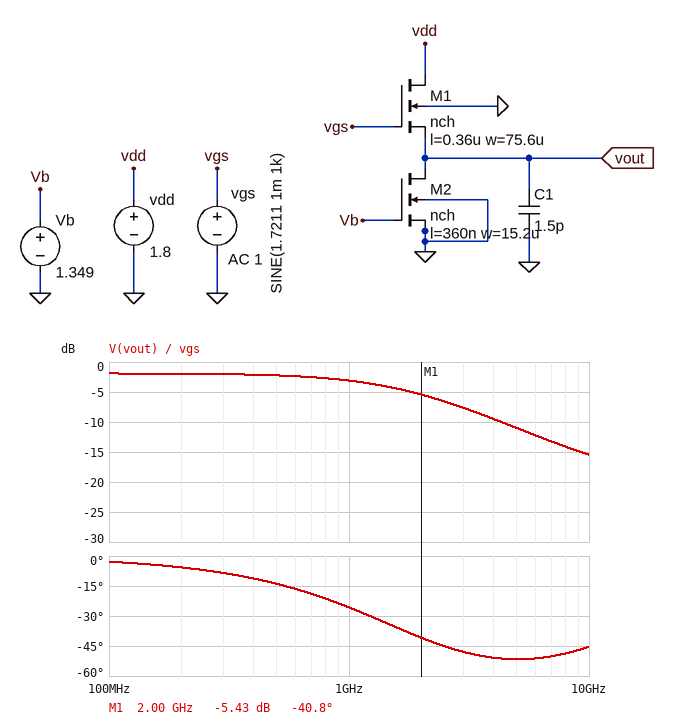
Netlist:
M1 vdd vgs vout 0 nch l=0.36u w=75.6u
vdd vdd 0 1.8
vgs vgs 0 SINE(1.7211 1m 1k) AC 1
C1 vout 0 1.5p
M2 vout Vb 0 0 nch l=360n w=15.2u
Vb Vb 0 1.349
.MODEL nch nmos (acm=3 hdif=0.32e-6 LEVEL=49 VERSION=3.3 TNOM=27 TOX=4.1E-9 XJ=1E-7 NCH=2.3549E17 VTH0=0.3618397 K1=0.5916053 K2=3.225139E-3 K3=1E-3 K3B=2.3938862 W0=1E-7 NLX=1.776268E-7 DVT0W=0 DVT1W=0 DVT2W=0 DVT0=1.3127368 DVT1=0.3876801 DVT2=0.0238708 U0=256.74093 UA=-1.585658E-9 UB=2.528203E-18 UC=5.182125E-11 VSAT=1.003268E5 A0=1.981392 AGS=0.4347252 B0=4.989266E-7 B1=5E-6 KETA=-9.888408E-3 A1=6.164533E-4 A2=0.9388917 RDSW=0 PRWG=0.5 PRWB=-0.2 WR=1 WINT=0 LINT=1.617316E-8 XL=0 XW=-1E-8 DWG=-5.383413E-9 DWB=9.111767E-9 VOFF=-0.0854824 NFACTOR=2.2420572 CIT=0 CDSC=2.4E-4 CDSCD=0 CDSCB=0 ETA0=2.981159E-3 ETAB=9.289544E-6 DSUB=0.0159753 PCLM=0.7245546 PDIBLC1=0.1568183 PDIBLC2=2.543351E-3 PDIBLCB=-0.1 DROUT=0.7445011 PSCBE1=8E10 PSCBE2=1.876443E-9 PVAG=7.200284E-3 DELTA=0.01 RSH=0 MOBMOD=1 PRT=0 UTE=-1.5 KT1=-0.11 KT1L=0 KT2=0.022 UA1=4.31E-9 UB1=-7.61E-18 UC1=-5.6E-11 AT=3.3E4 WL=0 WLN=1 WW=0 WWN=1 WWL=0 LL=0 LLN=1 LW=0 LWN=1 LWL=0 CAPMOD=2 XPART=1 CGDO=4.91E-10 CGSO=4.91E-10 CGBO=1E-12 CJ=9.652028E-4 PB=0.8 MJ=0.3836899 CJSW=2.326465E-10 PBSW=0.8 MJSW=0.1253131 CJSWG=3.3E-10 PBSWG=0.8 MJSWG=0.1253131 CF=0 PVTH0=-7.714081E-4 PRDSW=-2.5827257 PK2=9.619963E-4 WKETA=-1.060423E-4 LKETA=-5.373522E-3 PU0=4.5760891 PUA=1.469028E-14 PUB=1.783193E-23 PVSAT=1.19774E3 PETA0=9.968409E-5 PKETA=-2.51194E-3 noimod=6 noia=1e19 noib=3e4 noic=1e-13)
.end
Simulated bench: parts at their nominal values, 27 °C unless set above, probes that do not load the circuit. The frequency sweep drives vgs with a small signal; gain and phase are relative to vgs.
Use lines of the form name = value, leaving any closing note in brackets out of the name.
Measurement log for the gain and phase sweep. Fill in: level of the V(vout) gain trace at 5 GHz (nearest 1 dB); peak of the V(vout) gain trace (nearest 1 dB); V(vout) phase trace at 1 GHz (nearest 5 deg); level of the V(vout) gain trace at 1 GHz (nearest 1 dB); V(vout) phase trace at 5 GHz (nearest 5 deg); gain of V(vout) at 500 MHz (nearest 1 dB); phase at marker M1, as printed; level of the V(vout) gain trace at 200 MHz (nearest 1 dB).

level of the V(vout) gain trace at 5 GHz = -11 dB
peak of the V(vout) gain trace = -2 dB
V(vout) phase trace at 1 GHz = -25 deg
level of the V(vout) gain trace at 1 GHz = -3 dB
V(vout) phase trace at 5 GHz = -50 deg
gain of V(vout) at 500 MHz = -2 dB
phase at marker M1, as printed = -40.8 deg
level of the V(vout) gain trace at 200 MHz = -2 dB
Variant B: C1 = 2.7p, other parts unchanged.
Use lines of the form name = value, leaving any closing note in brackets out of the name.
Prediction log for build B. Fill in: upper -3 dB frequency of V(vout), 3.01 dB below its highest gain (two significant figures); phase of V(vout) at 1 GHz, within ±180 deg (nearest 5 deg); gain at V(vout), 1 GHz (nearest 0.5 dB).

upper -3 dB frequency of V(vout), 3.01 dB below its highest gain = 1.1 GHz
phase of V(vout) at 1 GHz, within ±180 deg = -40 deg
gain at V(vout), 1 GHz = -4.5 dB
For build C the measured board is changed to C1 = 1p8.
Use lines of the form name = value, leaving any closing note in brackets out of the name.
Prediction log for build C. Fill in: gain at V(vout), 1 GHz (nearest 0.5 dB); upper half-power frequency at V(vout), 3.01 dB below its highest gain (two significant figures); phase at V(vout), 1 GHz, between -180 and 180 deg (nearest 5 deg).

gain at V(vout), 1 GHz = -3.5 dB
upper half-power frequency at V(vout), 3.01 dB below its highest gain = 1.5 GHz
phase at V(vout), 1 GHz, between -180 and 180 deg = -30 deg
